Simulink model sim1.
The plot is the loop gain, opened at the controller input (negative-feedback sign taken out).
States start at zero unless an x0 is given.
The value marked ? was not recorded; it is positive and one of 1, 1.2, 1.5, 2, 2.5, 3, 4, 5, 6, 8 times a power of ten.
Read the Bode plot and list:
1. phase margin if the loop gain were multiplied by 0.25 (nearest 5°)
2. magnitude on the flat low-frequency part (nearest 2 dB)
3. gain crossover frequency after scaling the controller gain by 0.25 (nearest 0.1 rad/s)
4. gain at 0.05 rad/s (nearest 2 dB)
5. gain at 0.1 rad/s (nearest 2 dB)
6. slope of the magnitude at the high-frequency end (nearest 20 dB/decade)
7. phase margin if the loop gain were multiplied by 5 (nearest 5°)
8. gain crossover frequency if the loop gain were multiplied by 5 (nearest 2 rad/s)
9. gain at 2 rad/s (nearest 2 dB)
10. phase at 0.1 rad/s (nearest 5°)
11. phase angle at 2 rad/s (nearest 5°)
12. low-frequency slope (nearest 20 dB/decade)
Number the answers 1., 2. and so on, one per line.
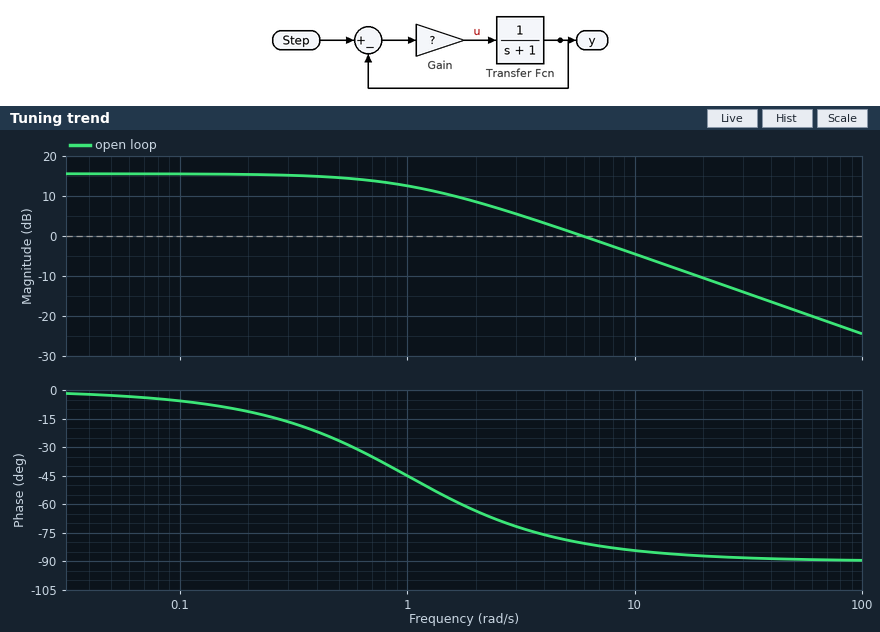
1. 130°
2. 16 dB
3. 1.1 rad/s
4. 16 dB
5. 16 dB
6. -20 dB/decade
7. 90°
8. 30 rad/s
9. 8 dB
10. -5°
11. -65°
12. 0 dB/decade
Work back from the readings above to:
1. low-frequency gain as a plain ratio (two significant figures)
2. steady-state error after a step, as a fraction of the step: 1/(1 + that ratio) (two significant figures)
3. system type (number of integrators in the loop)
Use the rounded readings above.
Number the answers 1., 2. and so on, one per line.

1. 6.3
2. 0.14
3. 0
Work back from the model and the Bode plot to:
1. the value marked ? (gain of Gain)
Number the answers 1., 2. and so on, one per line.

1. 6
